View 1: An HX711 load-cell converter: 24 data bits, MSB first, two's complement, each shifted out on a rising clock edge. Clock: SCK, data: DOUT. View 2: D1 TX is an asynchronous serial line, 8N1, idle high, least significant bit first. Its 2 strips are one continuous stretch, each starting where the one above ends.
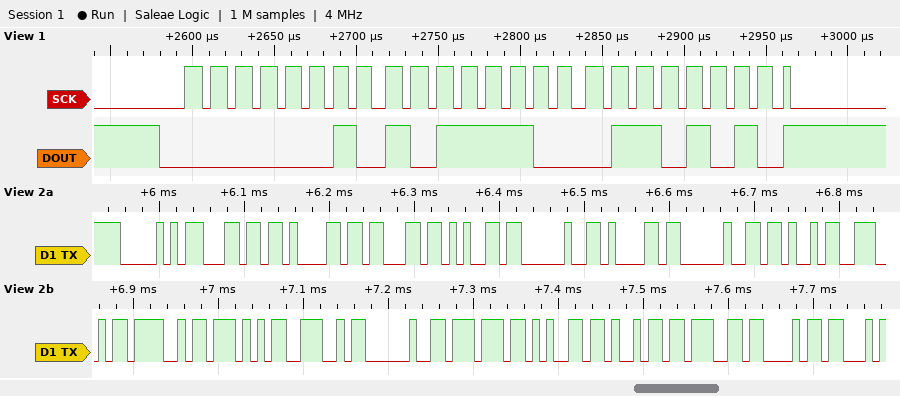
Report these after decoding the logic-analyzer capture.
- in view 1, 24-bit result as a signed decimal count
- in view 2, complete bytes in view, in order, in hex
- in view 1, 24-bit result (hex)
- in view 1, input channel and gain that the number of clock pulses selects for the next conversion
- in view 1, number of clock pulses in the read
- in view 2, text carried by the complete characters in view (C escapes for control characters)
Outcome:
179306
50 6C 61 63 65 20 61 20 4B 4E 4F 57 4E 20 77 65 69 67 68
0x02BC6A
channel A, gain 128
25
"Place a KNOWN weigh"
